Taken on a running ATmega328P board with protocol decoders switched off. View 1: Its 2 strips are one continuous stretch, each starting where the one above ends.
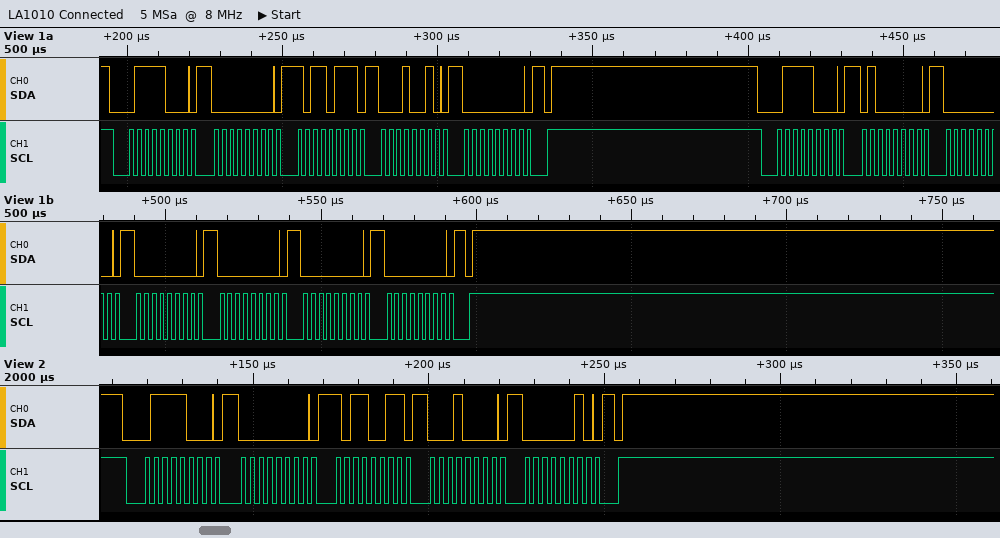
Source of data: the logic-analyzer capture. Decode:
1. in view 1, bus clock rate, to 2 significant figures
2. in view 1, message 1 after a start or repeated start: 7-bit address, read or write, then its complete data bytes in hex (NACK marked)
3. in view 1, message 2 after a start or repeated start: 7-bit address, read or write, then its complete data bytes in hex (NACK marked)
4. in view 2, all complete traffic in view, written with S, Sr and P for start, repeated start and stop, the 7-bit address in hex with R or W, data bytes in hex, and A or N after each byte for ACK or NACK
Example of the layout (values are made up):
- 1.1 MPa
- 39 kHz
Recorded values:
- 400 kHz
- 0x3C write: 00 B7 12 00
- 0x3C write: 40 00 00 00 00 00
- S 3CW A 00 A B3 A 10 A 02 A P
